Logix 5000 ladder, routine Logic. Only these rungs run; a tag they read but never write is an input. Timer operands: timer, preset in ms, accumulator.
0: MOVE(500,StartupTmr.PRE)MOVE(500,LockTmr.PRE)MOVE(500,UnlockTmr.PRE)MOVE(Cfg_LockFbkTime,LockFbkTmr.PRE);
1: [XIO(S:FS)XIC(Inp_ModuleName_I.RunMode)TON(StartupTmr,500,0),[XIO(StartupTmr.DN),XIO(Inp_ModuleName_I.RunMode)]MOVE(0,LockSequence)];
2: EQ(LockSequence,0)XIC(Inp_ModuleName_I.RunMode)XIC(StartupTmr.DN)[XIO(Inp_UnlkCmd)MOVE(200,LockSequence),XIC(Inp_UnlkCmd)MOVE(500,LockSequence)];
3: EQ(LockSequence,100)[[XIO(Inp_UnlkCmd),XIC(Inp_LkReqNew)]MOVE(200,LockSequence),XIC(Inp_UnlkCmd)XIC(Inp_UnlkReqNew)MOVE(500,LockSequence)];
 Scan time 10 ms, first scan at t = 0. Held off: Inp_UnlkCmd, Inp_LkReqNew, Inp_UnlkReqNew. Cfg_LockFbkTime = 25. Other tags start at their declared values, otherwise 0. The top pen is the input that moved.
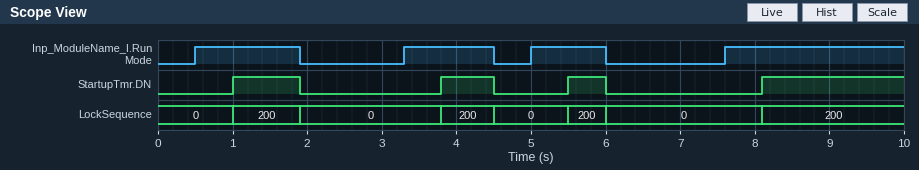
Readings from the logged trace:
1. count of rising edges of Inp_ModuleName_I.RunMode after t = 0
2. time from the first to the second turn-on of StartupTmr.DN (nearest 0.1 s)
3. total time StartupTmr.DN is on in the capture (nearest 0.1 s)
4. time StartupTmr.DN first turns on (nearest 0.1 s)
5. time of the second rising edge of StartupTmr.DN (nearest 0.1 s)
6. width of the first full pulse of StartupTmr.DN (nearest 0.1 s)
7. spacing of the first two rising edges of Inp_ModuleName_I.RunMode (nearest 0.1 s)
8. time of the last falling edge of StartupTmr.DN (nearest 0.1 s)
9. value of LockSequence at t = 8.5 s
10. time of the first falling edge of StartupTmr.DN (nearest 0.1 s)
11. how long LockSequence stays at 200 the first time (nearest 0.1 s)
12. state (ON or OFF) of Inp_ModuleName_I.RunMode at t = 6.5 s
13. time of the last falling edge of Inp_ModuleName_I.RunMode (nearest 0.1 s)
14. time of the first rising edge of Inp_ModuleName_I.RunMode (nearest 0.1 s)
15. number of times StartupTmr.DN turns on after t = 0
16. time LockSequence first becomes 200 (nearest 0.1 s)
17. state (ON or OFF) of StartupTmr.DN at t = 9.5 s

4
2.8 s
4.0 s
1.0 s
3.8 s
0.9 s
2.8 s
6.0 s
200
1.9 s
0.9 s
OFF
6.0 s
0.5 s
4
1.0 s
ON
